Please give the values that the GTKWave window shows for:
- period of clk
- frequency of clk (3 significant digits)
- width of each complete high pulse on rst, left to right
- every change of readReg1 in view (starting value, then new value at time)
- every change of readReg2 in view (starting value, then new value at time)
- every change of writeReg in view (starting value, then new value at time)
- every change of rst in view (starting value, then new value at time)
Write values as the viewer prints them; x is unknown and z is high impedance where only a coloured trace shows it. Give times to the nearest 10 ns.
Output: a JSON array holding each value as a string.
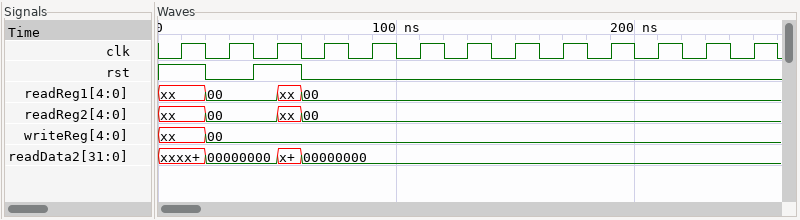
["20 ns", "50.0 MHz", "20 ns", "xx, 00 at 20 ns, xx at 50 ns, 00 at 60 ns", "xx, 00 at 20 ns, xx at 50 ns, 00 at 60 ns", "xx, 00 at 20 ns", "1, 0 at 20 ns, 1 at 40 ns, 0 at 60 ns"]
